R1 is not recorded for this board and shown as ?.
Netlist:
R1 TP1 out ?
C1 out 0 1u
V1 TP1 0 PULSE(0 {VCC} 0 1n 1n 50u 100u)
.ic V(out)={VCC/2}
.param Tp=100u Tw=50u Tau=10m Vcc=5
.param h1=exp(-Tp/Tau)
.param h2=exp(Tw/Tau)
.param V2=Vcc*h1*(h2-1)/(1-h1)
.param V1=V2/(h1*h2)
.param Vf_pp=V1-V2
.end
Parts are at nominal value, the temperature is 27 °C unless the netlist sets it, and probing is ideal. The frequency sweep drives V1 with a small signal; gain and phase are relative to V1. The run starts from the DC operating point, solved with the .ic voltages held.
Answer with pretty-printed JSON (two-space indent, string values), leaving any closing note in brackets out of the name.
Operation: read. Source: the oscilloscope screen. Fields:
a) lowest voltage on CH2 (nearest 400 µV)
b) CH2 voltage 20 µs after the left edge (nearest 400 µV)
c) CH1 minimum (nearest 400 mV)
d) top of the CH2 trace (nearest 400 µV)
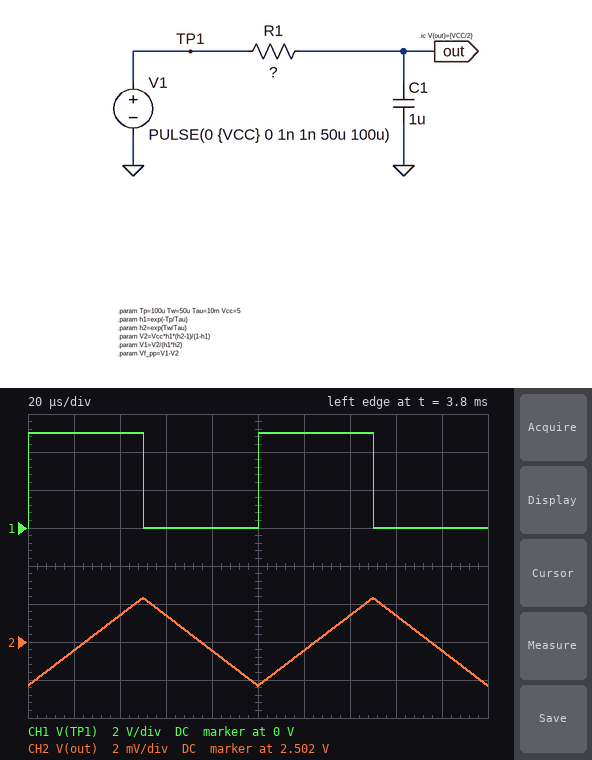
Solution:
{
  "lowest voltage on CH2": "2.4996 V",
  "CH2 voltage 20 µs after the left edge": "2.5016 V",
  "CH1 minimum": "0 V",
  "top of the CH2 trace": "2.5044 V"
}
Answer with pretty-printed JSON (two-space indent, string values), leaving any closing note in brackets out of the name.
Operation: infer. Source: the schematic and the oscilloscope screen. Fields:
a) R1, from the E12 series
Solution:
{
  "R1, from the E12 series": "27 kΩ"
}
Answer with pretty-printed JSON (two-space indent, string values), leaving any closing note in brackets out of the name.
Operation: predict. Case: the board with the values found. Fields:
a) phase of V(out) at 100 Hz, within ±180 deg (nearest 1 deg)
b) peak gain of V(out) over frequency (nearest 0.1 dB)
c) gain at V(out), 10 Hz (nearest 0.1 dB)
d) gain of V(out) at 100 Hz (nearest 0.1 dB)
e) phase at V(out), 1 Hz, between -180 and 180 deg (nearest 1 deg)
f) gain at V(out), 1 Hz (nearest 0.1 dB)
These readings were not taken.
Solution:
{
  "phase of V(out) at 100 Hz, within ±180 deg": "-87 deg",
  "peak gain of V(out) over frequency": "0 dB",
  "gain at V(out), 10 Hz": "-5.9 dB",
  "gain of V(out) at 100 Hz": "-24.6 dB",
  "phase at V(out), 1 Hz, between -180 and 180 deg": "-10 deg",
  "gain at V(out), 1 Hz": "-0.1 dB"
}
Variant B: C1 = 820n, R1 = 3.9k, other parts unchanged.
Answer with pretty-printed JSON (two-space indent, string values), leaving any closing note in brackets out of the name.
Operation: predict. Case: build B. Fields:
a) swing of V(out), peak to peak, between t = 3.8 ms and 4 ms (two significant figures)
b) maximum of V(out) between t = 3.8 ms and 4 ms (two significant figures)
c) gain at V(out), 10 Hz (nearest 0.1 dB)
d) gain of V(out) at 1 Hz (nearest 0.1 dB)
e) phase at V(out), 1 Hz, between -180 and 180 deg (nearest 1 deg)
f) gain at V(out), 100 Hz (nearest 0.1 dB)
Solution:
{
  "swing of V(out), peak to peak, between t = 3.8 ms and 4 ms": "39 mV",
  "maximum of V(out) between t = 3.8 ms and 4 ms": "2.5 V",
  "gain at V(out), 10 Hz": "-0.2 dB",
  "gain of V(out) at 1 Hz": "0 dB",
  "phase at V(out), 1 Hz, between -180 and 180 deg": "-1 deg",
  "gain at V(out), 100 Hz": "-7.0 dB"
}
